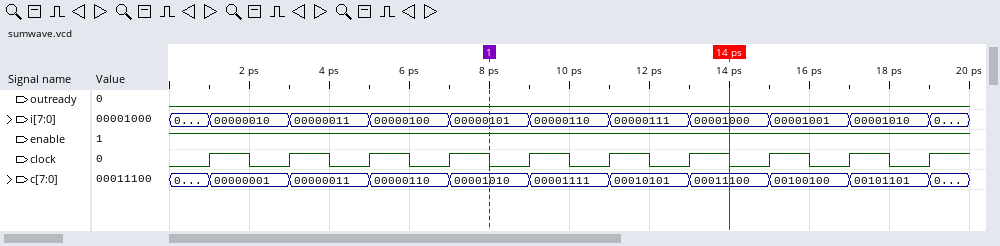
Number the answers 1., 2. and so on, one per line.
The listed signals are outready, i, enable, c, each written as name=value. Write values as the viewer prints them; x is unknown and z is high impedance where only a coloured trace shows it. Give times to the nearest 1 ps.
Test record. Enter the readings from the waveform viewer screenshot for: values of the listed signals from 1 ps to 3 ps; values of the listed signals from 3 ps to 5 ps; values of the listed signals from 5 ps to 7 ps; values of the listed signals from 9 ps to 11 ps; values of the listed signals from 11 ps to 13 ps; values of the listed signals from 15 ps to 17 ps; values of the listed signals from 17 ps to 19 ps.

1. outready=0, i=00000010, enable=1, c=00000001
2. outready=0, i=00000011, enable=1, c=00000011
3. outready=0, i=00000100, enable=1, c=00000110
4. outready=0, i=00000110, enable=1, c=00001111
5. outready=0, i=00000111, enable=1, c=00010101
6. outready=0, i=00001001, enable=1, c=00100100
7. outready=0, i=00001010, enable=1, c=00101101
